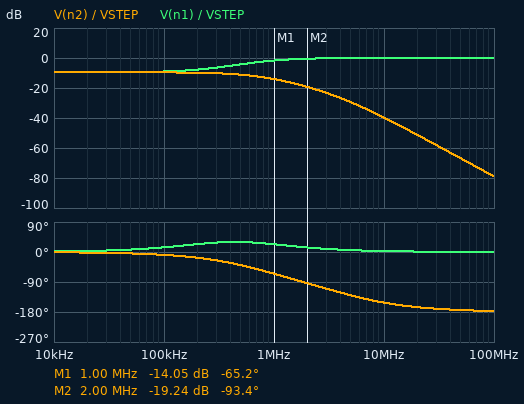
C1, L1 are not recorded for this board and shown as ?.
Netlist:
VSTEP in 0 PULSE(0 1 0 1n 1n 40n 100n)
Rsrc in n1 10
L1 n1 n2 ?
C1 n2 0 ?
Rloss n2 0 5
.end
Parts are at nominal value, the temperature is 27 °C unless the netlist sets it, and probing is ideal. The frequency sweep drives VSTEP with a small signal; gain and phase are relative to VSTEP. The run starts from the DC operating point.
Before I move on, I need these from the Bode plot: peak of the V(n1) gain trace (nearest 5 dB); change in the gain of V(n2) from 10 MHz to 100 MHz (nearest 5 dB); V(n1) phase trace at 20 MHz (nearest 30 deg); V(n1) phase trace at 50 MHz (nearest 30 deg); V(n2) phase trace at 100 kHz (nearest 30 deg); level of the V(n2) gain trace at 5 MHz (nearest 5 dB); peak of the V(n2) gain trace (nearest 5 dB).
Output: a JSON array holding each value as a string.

["0 dB", "-40 dB", "0 deg", "0 deg", "0 deg", "-30 dB", "-10 dB"]
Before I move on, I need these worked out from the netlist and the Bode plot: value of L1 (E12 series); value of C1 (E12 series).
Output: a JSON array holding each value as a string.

["3.3 µH", "6.8 nF"]
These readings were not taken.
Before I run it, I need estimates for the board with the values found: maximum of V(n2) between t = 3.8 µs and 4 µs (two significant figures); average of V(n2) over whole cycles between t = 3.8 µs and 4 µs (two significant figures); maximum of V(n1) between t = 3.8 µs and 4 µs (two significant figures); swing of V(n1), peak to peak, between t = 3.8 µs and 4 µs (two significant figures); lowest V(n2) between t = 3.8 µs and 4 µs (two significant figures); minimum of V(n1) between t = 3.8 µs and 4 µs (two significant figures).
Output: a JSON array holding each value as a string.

["140 mV", "140 mV", "760 mV", "1.1 V", "130 mV", "-310 mV"]
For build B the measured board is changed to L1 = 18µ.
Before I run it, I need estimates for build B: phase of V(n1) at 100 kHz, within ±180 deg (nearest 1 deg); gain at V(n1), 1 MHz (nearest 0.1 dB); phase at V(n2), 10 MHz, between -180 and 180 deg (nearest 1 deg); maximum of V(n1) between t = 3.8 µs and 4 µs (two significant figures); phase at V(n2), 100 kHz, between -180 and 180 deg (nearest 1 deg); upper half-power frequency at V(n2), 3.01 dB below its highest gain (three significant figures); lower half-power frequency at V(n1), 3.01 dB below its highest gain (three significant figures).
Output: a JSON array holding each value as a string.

["29 deg", "-0.1 dB", "-154 deg", "740 mV", "-38 deg", "134 kHz", "118 kHz"]
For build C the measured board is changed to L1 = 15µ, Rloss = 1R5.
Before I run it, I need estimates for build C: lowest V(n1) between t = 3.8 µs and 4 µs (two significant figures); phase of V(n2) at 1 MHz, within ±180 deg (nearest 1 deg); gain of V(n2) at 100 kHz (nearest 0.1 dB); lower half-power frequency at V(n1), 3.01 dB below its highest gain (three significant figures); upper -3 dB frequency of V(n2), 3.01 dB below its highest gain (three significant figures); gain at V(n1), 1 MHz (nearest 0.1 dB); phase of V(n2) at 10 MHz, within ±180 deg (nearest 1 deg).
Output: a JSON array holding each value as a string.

["-350 mV", "-87 deg", "-19.9 dB", "120 kHz", "122 kHz", "-0.1 dB", "-122 deg"]
